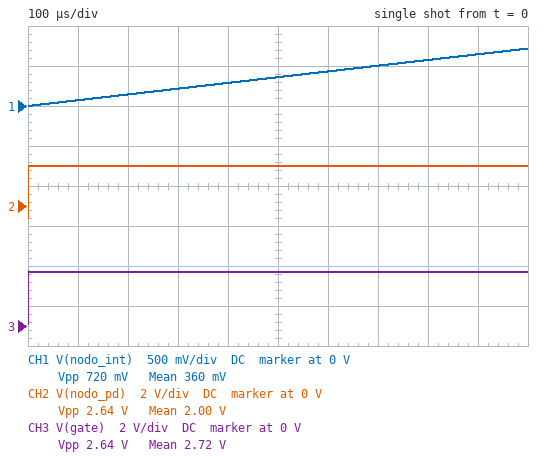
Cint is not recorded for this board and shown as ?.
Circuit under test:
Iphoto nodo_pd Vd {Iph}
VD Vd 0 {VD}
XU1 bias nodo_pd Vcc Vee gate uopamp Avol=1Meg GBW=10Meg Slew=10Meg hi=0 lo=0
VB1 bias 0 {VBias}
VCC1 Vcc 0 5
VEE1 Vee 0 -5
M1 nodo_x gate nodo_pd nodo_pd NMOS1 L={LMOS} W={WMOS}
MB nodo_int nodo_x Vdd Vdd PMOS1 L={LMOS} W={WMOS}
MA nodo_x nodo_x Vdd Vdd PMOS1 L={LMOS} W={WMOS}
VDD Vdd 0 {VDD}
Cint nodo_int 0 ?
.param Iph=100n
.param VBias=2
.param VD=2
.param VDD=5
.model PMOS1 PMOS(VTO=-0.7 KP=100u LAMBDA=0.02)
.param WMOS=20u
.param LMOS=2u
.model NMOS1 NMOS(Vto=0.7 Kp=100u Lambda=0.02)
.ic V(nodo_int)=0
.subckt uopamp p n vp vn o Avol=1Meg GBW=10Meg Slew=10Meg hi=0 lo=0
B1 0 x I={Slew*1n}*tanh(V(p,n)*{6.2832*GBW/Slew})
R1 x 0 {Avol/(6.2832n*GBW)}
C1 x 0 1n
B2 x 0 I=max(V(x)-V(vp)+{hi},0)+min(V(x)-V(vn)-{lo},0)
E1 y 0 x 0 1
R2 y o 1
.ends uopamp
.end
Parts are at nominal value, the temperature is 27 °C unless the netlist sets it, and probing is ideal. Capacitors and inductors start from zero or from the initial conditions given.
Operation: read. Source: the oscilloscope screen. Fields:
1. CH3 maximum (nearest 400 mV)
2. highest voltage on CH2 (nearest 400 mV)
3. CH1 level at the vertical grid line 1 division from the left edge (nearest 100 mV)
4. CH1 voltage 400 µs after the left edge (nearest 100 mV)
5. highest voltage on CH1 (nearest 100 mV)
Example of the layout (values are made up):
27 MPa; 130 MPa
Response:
2.8 V; 2.0 V; 100 mV; 300 mV; 700 mV
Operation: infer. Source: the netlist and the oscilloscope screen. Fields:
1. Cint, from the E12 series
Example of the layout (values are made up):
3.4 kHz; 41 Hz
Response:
150 pF
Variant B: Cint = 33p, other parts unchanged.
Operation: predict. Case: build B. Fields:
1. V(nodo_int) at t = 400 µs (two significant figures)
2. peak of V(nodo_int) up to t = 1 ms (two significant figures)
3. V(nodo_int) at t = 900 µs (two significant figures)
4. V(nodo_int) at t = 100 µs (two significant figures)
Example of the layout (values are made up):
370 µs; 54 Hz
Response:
1.3 V; 3.2 V; 2.9 V; 330 mV
